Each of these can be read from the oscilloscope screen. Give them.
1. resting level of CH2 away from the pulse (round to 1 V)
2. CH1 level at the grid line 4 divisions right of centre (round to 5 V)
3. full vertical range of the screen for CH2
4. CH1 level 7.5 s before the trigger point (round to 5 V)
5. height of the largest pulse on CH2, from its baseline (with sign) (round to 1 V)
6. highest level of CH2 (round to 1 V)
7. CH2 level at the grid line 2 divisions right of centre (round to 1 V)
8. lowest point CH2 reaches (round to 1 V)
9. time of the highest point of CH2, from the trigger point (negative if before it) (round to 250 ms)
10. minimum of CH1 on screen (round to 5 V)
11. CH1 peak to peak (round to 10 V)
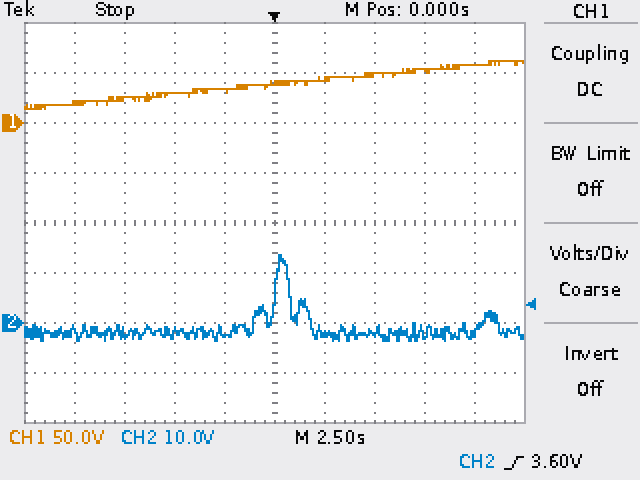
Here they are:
-2 V
60 V
80 V
25 V
+16 V
14 V
-2 V
-4 V
+250 ms
15 V
50 V
